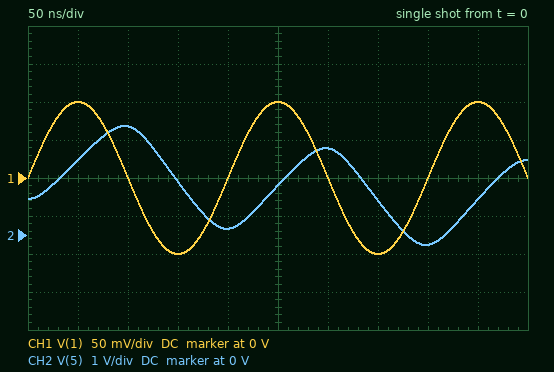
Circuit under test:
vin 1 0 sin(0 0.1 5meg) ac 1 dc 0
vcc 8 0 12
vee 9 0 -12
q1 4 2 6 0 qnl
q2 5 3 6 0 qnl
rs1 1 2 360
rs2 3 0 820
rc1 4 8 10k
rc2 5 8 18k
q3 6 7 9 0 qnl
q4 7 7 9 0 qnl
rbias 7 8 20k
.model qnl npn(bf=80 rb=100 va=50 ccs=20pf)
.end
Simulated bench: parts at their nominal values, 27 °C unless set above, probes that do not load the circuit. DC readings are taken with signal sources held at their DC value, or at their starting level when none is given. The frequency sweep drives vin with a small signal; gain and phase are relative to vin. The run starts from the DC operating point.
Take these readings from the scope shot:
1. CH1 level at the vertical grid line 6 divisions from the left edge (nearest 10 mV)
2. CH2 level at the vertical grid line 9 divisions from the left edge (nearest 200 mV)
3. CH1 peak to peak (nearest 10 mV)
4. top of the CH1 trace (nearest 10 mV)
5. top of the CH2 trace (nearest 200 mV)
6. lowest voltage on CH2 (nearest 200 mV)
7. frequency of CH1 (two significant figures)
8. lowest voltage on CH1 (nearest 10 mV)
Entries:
0 V
1.0 V
200 mV
100 mV
2.8 V
-200 mV
5.0 MHz
-100 mV
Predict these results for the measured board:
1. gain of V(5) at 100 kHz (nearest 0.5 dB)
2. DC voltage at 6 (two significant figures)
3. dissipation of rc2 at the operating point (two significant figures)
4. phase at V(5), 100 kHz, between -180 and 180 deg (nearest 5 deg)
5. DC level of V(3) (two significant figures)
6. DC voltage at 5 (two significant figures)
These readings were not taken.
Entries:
44.0 dB
-770 mV
6.8 mW
-10 deg
-6.2 mV
950 mV
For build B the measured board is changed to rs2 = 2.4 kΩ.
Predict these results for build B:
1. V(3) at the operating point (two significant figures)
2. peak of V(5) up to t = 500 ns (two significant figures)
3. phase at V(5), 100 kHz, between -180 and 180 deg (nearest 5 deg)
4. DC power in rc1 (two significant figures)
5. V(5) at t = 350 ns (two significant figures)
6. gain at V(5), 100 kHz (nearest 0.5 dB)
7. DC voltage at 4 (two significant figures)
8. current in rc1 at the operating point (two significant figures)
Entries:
-15 mV
4.1 V
-10 deg
6.9 mW
2.1 V
42.5 dB
3.7 V
830 µA
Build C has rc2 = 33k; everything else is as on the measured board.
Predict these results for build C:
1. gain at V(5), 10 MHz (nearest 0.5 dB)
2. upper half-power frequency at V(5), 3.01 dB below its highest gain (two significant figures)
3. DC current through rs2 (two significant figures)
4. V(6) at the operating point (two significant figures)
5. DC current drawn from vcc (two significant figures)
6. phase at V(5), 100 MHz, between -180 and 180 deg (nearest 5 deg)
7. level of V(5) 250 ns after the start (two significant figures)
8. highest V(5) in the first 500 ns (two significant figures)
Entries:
5.5 dB
38 MHz
26 µA
-780 mV
2.5 mA
-85 deg
-110 mV
410 mV
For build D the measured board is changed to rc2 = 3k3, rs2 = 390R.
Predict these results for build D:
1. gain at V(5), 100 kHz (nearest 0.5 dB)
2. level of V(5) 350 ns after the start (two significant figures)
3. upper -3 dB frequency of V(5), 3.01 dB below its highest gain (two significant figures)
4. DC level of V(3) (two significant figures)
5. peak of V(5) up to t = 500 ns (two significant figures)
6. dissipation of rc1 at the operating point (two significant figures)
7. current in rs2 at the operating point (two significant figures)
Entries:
31.0 dB
9.3 V
2.7 MHz
-2.9 mV
11 V
4.3 mW
7.3 µA
